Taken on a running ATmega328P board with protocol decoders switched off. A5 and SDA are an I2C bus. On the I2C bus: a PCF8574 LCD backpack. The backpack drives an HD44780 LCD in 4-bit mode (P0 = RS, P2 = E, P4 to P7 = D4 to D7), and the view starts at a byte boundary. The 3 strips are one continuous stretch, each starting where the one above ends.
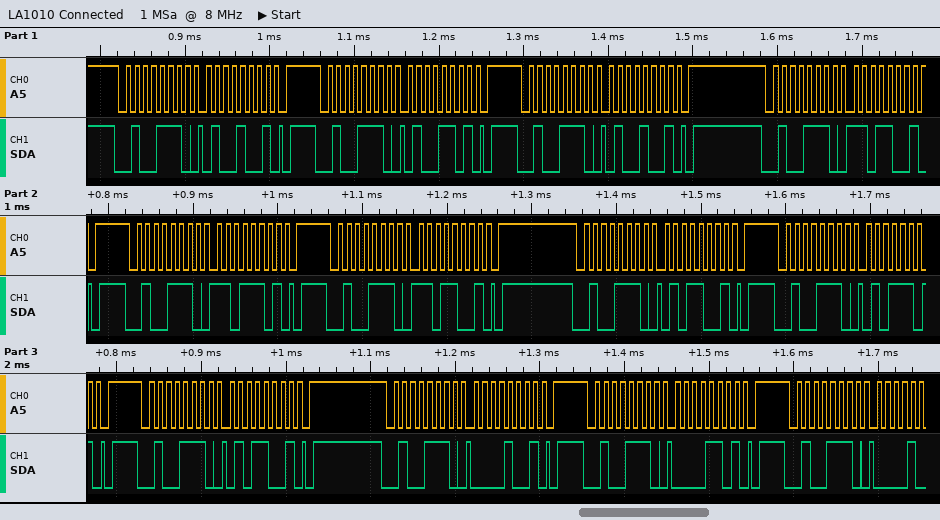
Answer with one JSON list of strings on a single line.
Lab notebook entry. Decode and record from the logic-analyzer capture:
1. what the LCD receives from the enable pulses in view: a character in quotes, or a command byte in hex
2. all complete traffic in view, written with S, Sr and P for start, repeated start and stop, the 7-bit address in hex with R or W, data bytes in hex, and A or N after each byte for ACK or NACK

["'M'", "S 27W A 49 A P S 27W A 4D A P S 27W A 49 A P S 27W A D9 A P S 27W A DD A P S 27W A D9 A P S 27W A 59 A P S 27W A 5D A P S 27W A 59 A P S 27W A 09 A P S 27W A 0D A P S 27W A"]
